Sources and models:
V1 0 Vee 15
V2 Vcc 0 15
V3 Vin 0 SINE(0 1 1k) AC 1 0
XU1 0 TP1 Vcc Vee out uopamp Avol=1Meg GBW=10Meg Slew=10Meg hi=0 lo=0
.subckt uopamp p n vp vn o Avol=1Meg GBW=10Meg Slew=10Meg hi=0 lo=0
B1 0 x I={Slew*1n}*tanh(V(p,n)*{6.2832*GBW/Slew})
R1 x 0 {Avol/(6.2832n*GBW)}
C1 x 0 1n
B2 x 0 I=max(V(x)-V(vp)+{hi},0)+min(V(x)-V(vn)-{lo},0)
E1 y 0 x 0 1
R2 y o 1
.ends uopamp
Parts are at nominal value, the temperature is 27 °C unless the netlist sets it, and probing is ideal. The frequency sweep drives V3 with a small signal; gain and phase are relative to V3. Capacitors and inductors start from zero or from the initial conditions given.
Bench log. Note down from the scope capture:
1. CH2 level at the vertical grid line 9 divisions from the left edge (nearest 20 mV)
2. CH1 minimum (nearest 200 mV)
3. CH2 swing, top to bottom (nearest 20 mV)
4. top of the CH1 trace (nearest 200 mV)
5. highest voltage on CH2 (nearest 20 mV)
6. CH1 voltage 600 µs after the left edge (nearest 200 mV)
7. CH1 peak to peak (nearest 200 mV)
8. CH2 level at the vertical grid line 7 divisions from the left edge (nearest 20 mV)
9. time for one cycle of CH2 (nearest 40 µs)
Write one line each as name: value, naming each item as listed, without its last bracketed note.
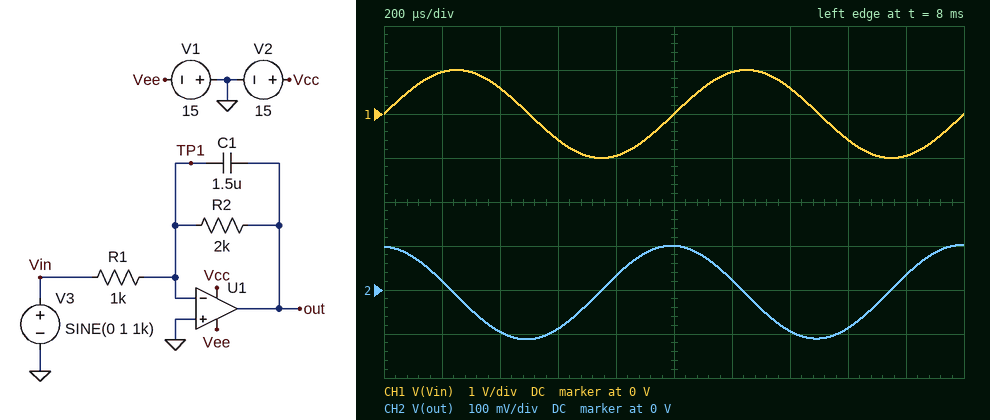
CH2 level at the vertical grid line 9 divisions from the left edge: 40 mV
CH1 minimum: -1.0 V
CH2 swing, top to bottom: 220 mV
top of the CH1 trace: 1.0 V
highest voltage on CH2: 100 mV
CH1 voltage 600 µs after the left edge: -600 mV
CH1 peak to peak: 2.0 V
CH2 level at the vertical grid line 7 divisions from the left edge: -100 mV
time for one cycle of CH2: 1.00 ms
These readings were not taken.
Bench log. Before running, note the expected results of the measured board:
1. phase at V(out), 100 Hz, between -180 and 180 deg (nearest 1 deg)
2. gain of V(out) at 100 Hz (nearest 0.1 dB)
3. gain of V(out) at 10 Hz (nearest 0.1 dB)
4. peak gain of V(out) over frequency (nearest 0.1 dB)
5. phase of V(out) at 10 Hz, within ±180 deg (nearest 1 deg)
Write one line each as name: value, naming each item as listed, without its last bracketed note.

phase at V(out), 100 Hz, between -180 and 180 deg: 118 deg
gain of V(out) at 100 Hz: -0.6 dB
gain of V(out) at 10 Hz: 5.9 dB
peak gain of V(out) over frequency: 6.0 dB
phase of V(out) at 10 Hz, within ±180 deg: 169 deg
